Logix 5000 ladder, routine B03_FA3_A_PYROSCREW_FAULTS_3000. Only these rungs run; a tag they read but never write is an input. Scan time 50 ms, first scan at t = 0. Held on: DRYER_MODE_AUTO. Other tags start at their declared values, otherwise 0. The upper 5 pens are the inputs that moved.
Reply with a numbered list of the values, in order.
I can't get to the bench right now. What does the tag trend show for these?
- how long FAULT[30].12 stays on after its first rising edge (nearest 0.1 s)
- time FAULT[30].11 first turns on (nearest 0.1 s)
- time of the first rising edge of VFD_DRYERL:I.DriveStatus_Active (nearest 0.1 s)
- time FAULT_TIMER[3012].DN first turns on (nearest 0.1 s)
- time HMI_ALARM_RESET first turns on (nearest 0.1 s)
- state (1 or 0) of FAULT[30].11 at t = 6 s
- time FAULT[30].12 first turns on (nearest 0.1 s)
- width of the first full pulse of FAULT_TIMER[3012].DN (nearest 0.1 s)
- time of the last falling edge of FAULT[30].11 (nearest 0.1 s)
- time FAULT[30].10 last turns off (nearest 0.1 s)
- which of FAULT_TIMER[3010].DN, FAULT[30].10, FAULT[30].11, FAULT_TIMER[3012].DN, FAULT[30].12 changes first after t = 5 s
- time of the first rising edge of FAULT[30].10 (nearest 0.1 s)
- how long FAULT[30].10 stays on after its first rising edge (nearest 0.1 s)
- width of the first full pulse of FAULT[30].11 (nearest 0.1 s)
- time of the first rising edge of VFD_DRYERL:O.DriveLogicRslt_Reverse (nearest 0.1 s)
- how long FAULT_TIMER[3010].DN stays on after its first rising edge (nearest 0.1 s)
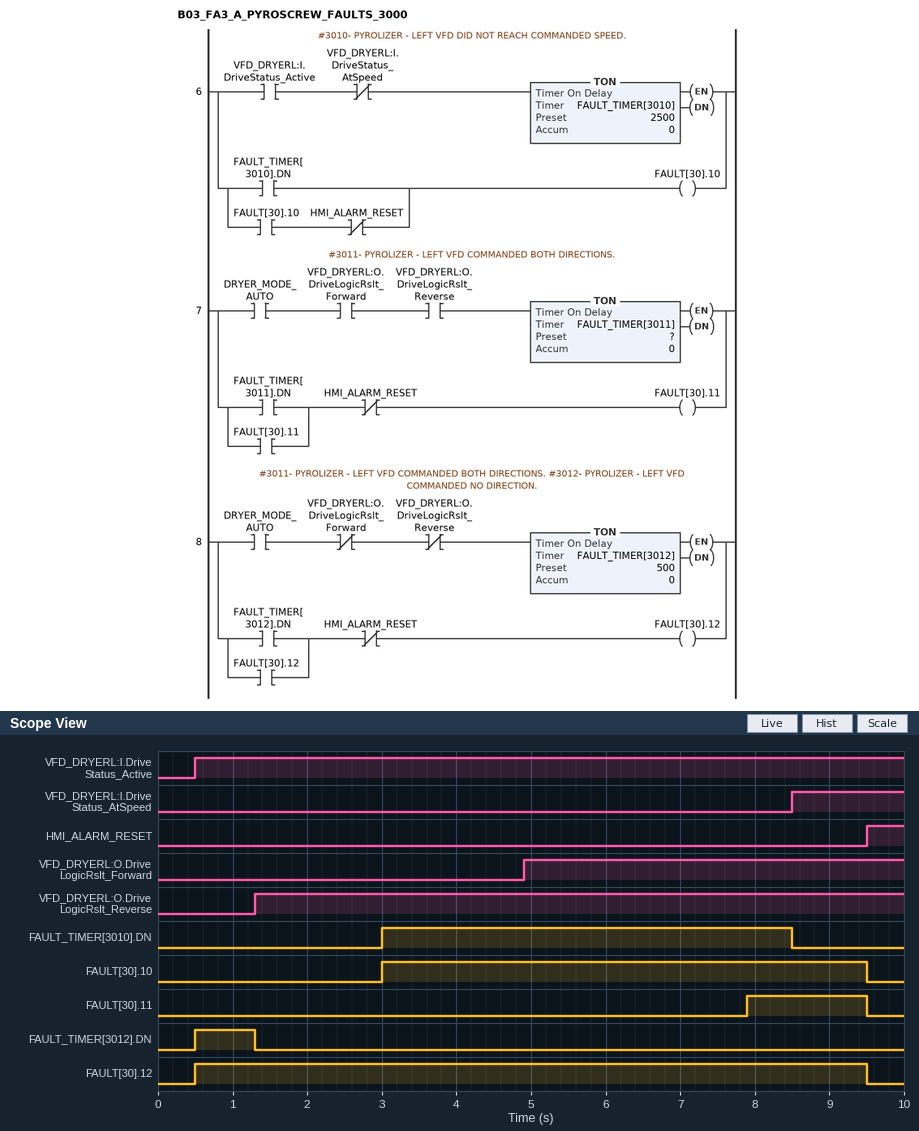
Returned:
1. 9.0 s
2. 7.9 s
3. 0.5 s
4. 0.5 s
5. 9.5 s
6. 0
7. 0.5 s
8. 0.8 s
9. 9.5 s
10. 9.5 s
11. FAULT[30].11
12. 3.0 s
13. 6.5 s
14. 1.6 s
15. 1.3 s
16. 5.5 s
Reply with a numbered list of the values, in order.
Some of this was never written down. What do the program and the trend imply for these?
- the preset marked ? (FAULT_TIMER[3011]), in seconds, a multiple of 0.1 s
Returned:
1. 3.0 s
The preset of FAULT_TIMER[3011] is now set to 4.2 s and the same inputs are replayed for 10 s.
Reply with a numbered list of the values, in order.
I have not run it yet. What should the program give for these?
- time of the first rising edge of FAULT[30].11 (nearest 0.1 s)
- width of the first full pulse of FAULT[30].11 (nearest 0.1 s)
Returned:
1. 9.1 s
2. 0.4 s
